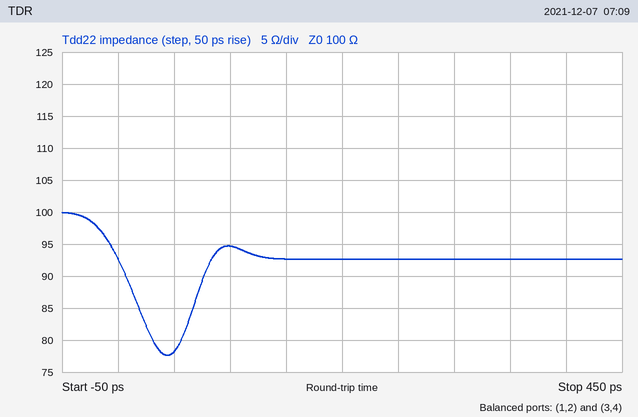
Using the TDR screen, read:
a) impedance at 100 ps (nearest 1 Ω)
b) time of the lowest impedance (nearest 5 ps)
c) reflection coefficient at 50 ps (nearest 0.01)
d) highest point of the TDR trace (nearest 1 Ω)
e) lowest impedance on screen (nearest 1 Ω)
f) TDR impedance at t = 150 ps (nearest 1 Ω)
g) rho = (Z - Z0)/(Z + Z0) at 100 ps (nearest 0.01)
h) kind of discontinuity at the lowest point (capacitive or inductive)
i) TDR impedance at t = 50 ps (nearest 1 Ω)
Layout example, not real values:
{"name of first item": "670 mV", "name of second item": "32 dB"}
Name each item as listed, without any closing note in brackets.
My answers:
{"impedance at 100 ps": "95 Ω", "time of the lowest impedance": "45 ps", "reflection coefficient at 50 ps": "-0.12", "highest point of the TDR trace": "100 Ω", "lowest impedance on screen": "78 Ω", "TDR impedance at t = 150 ps": "93 Ω", "rho = (Z - Z0)/(Z + Z0) at 100 ps": "-0.03", "kind of discontinuity at the lowest point": "capacitive", "TDR impedance at t = 50 ps": "78 Ω"}
